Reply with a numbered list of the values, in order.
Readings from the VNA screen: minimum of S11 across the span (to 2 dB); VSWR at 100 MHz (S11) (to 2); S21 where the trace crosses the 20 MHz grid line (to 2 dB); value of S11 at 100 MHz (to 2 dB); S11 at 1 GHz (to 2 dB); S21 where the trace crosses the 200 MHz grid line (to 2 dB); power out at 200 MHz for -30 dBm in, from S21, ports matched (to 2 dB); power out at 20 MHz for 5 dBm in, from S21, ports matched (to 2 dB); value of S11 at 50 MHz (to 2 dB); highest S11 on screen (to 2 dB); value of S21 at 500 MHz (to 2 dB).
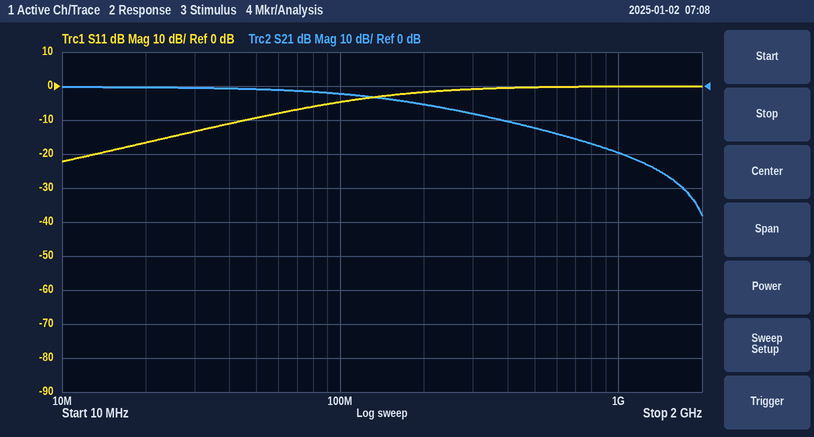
1. -22 dB
2. 4
3. 0 dB
4. -4 dB
5. 0 dB
6. -6 dB
7. -36 dBm
8. 4 dBm
9. -10 dB
10. 0 dB
11. -12 dB
